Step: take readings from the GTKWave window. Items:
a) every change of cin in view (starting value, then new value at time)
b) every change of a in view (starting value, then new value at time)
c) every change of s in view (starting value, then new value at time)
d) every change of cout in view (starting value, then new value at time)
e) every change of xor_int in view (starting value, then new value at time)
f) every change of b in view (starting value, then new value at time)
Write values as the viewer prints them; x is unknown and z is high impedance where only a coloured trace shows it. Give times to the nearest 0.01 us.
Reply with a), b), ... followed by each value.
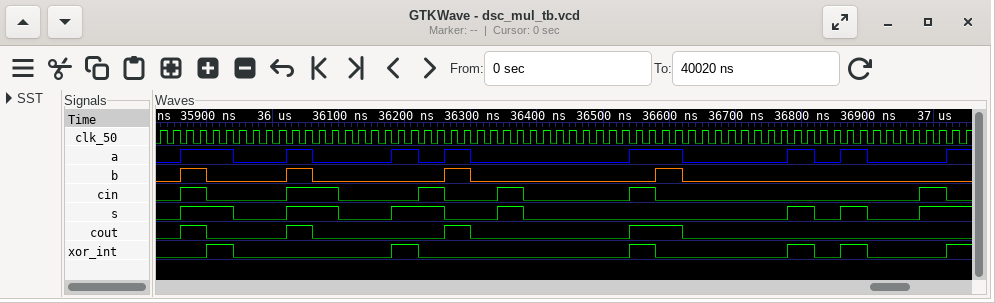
a) 0, 1 at 35.86 us, 0 at 35.9 us, 1 at 36.02 us, 0 at 36.1 us, 1 at 36.22 us, 0 at 36.26 us, 1 at 36.34 us, 0 at 36.38 us, 1 at 36.54 us, 0 at 36.58 us, 1 at 36.98 us, 0 at 37.02 us
b) 0, 1 at 35.86 us, 0 at 35.94 us, 1 at 36.02 us, 0 at 36.06 us, 1 at 36.18 us, 0 at 36.22 us, 1 at 36.26 us, 0 at 36.3 us, 1 at 36.54 us, 0 at 36.62 us, 1 at 36.78 us, 0 at 36.82 us, 1 at 36.86 us, 0 at 36.9 us, 1 at 37.02 us
c) 0, 1 at 35.86 us, 0 at 35.94 us, 1 at 36.02 us, 0 at 36.1 us, 1 at 36.18 us, 0 at 36.26 us, 1 at 36.34 us, 0 at 36.38 us, 1 at 36.78 us, 0 at 36.82 us, 1 at 36.86 us, 0 at 36.9 us, 1 at 36.98 us
d) 0, 1 at 35.86 us, 0 at 35.9 us, 1 at 36.02 us, 0 at 36.06 us, 1 at 36.26 us, 0 at 36.3 us, 1 at 36.54 us, 0 at 36.62 us
e) 0, 1 at 35.9 us, 0 at 35.94 us, 1 at 36.18 us, 0 at 36.22 us, 1 at 36.54 us, 0 at 36.58 us, 1 at 36.78 us, 0 at 36.82 us, 1 at 36.86 us, 0 at 36.9 us, 1 at 37.02 us
f) 0, 1 at 35.86 us, 0 at 35.9 us, 1 at 36.02 us, 0 at 36.06 us, 1 at 36.26 us, 0 at 36.3 us, 1 at 36.58 us, 0 at 36.62 us
